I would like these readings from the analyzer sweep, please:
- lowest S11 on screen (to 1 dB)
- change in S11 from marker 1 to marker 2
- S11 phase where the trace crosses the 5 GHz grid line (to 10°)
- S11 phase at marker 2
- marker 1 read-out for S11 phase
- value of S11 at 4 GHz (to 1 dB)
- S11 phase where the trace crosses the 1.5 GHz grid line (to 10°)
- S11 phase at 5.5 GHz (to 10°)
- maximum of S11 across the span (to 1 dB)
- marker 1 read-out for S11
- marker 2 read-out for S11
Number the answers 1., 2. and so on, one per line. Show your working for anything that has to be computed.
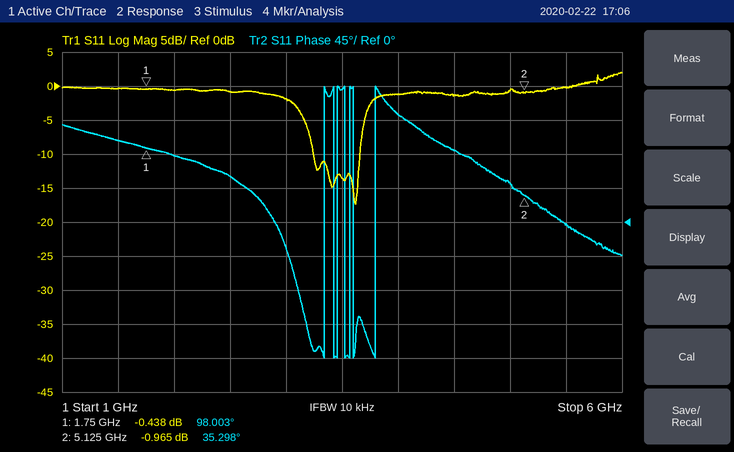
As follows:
1. -17 dB
2. -0.965 − (-0.438) = -0.527 dB
3. 50°
4. 35.298°
5. 98.003°
6. -1 dB
7. 110°
8. 0°
9. 2 dB
10. -0.438 dB
11. -0.965 dB
